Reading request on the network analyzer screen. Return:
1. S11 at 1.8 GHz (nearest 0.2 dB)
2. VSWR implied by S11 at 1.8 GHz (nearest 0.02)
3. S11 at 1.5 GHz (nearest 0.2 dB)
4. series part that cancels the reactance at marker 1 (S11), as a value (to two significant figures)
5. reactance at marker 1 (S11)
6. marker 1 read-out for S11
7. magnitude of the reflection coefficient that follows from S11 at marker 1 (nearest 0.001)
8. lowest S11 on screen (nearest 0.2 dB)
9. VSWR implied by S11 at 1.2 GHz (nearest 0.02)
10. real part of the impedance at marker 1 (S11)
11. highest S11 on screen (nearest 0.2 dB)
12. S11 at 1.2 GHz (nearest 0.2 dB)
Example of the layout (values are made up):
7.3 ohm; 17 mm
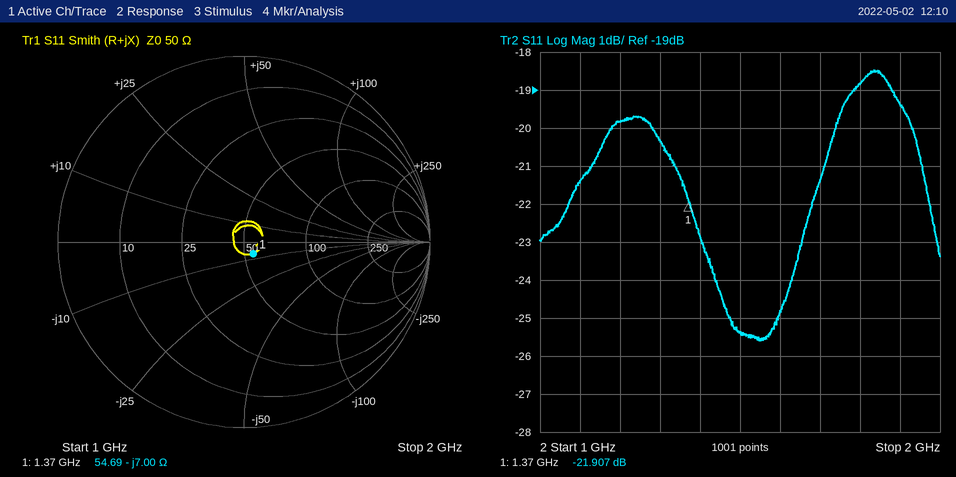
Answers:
-18.8 dB; 1.26; -25.4 dB; 810 pH; -7.00 Ω; -21.907 dB; 0.080; -25.6 dB; 1.22; 54.69 Ω; -18.4 dB; -19.8 dB
